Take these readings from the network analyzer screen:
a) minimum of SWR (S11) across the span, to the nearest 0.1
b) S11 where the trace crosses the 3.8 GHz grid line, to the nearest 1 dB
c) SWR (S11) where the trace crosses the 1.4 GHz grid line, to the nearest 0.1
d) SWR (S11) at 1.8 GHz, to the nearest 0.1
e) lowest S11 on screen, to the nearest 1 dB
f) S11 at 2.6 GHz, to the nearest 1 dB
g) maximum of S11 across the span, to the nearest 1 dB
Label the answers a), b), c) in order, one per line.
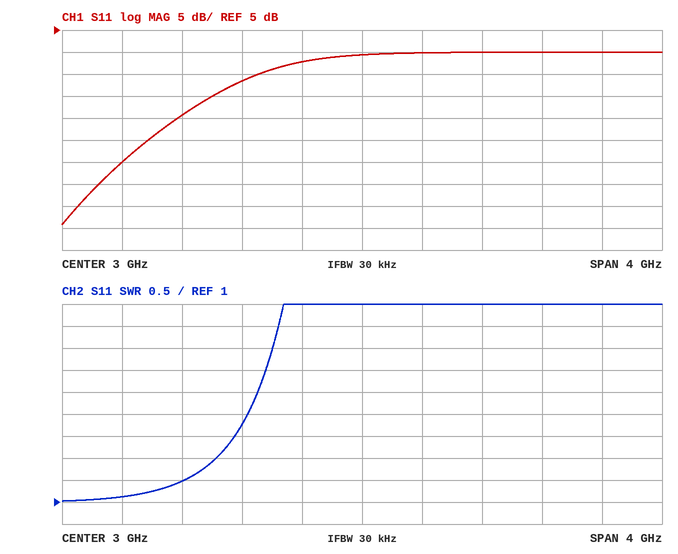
a) 1.0
b) 0 dB
c) 1.1
d) 1.5
e) -39 dB
f) -2 dB
g) 0 dB
